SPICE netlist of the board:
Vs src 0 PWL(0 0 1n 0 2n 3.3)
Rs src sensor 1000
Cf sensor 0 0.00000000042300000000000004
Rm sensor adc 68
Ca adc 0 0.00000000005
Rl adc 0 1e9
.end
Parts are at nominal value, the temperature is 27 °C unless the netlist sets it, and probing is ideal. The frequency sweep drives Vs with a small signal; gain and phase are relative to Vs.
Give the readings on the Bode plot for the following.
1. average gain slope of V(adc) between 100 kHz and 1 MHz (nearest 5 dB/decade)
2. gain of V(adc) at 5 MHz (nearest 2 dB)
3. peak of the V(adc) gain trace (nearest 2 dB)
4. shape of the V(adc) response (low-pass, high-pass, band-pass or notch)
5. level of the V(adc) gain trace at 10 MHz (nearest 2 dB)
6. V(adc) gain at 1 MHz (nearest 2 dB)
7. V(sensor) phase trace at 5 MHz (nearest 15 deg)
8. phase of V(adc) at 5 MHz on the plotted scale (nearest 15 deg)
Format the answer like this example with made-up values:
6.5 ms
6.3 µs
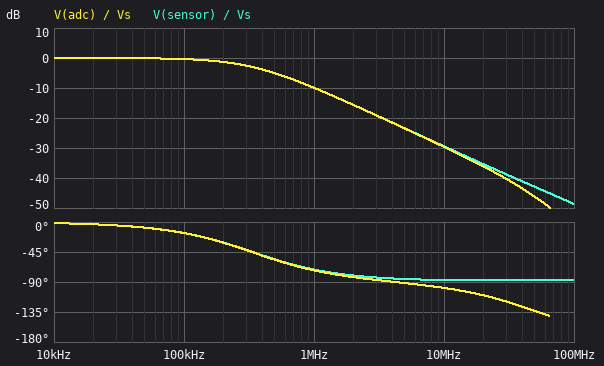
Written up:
-10 dB/decade
-24 dB
0 dB
low-pass
-30 dB
-10 dB
-90 deg
-90 deg
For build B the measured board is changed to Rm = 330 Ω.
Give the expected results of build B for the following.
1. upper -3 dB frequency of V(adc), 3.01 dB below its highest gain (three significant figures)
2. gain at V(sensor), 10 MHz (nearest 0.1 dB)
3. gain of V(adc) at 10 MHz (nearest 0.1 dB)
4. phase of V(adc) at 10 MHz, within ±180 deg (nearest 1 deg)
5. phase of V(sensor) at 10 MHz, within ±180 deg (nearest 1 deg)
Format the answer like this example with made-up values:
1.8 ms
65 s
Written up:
335 kHz
-29.0 dB
-32.2 dB
-131 deg
-85 deg
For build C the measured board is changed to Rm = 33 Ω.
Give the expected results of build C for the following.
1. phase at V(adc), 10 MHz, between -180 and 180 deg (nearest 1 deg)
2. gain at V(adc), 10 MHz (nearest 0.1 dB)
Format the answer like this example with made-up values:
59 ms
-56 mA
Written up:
-93 deg
-29.5 dB
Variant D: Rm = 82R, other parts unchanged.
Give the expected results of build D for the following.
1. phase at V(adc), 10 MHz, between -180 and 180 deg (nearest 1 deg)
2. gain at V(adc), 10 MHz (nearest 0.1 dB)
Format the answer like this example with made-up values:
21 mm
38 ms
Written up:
-101 deg
-29.7 dB
